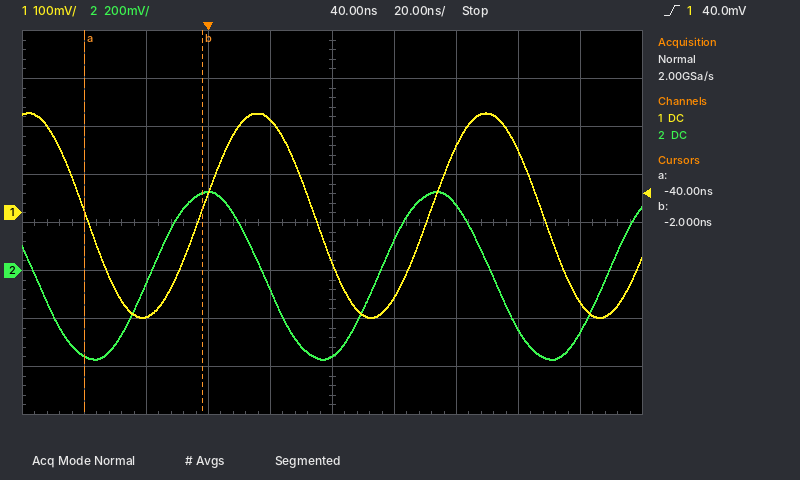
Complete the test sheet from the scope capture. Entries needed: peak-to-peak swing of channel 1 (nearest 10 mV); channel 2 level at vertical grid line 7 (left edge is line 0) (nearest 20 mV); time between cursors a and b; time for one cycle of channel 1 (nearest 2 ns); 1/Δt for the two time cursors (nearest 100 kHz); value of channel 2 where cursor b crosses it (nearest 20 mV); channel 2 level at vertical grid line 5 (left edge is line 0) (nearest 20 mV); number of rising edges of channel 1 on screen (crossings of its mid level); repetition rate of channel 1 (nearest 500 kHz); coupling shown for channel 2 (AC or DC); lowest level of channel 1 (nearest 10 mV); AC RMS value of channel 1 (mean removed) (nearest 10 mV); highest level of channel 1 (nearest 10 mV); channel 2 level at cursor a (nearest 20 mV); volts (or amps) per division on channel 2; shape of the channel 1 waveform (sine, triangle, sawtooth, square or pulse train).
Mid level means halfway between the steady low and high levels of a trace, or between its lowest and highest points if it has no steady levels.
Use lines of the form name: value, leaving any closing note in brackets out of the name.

peak-to-peak swing of channel 1: 430 mV
channel 2 level at vertical grid line 7 (left edge is line 0): 280 mV
time between cursors a and b: 38 ns
time for one cycle of channel 1: 74 ns
1/Δt for the two time cursors: 26.3 MHz
value of channel 2 where cursor b crosses it: 320 mV
channel 2 level at vertical grid line 5 (left edge is line 0): -360 mV
number of rising edges of channel 1 on screen: 2
repetition rate of channel 1: 13.5 MHz
coupling shown for channel 2: DC
lowest level of channel 1: -220 mV
AC RMS value of channel 1 (mean removed): 150 mV
highest level of channel 1: 210 mV
channel 2 level at cursor a: -360 mV
volts (or amps) per division on channel 2: 200 mV
shape of the channel 1 waveform: sine
